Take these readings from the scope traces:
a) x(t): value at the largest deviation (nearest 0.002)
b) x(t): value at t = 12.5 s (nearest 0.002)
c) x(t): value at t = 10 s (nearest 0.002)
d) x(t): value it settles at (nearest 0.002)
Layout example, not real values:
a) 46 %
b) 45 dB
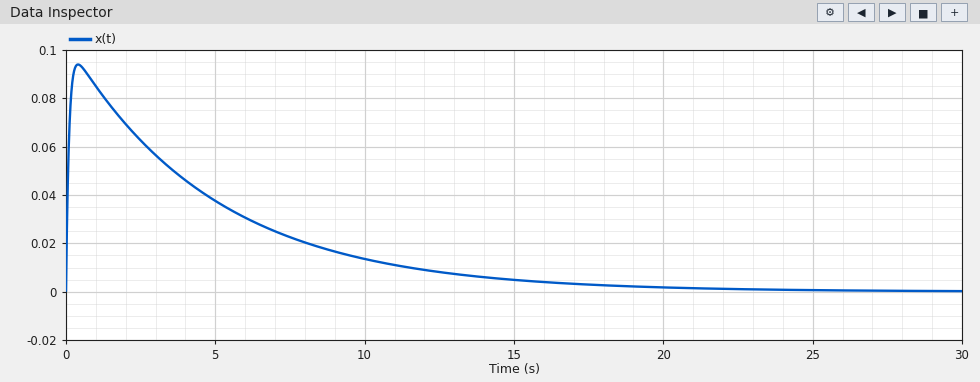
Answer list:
a) 0.094
b) 0.008
c) 0.014
d) 0.000
